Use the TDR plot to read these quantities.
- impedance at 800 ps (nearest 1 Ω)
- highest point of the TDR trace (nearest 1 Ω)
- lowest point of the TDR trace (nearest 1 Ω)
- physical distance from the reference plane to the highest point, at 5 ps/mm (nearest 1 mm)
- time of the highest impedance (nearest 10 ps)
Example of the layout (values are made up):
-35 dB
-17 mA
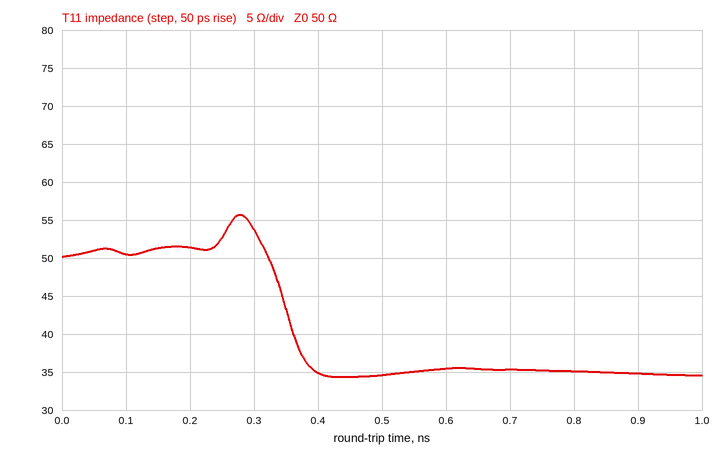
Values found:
35 Ω
56 Ω
34 Ω
28 mm
280 ps
